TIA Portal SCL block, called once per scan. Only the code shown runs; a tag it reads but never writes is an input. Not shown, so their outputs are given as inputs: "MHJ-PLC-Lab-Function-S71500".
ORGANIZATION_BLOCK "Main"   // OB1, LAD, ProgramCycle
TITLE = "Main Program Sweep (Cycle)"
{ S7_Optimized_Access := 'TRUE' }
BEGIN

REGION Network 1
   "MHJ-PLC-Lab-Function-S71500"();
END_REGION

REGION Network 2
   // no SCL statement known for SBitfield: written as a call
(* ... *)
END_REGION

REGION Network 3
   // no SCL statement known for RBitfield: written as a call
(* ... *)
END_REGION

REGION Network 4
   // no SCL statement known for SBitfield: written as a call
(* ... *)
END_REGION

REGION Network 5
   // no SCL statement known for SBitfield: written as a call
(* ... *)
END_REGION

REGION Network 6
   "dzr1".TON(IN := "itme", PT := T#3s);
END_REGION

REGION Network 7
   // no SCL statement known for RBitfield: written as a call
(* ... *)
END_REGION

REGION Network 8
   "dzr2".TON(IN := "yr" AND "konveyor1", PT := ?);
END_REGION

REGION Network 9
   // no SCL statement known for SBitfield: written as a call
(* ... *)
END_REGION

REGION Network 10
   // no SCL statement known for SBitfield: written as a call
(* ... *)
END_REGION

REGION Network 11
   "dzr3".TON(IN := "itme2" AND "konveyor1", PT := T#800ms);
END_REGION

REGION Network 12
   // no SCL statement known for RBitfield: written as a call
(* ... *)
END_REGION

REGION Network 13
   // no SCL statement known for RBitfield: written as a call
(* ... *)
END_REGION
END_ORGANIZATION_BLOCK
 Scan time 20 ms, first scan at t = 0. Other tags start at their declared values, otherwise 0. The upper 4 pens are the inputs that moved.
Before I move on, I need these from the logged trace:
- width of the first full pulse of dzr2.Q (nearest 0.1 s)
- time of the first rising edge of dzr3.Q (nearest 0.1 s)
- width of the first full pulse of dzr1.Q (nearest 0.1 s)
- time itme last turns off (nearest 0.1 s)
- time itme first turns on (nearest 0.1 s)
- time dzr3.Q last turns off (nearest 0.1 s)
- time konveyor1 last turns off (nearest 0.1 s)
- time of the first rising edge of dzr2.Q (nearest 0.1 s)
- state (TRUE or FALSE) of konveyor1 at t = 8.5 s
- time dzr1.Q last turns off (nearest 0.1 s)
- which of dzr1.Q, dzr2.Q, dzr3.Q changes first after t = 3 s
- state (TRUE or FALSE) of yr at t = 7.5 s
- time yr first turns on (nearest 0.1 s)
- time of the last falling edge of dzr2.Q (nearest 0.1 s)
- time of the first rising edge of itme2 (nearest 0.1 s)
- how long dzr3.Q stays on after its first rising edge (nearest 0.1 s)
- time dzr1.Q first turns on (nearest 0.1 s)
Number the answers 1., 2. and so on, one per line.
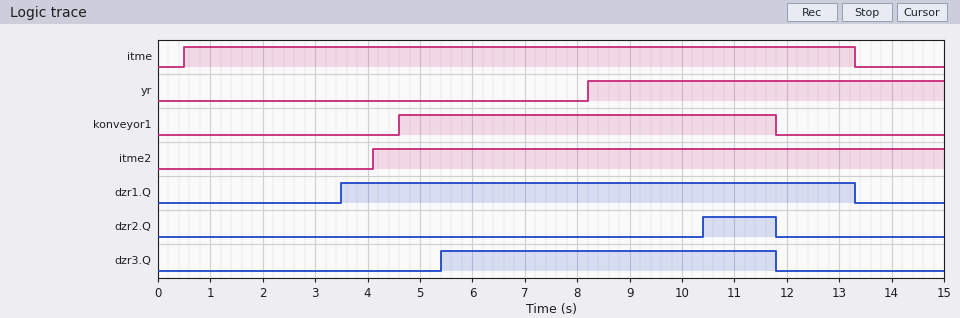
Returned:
1. 1.4 s
2. 5.4 s
3. 9.8 s
4. 13.3 s
5. 0.5 s
6. 11.8 s
7. 11.8 s
8. 10.4 s
9. TRUE
10. 13.3 s
11. dzr1.Q
12. FALSE
13. 8.2 s
14. 11.8 s
15. 4.1 s
16. 6.4 s
17. 3.5 s
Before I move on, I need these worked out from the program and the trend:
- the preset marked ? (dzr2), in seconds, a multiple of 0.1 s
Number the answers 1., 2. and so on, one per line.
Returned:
1. 2.2 s
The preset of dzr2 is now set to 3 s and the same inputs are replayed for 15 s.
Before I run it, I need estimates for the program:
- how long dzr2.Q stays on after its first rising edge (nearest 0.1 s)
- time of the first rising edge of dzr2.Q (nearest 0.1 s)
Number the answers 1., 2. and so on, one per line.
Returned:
1. 0.6 s
2. 11.2 s
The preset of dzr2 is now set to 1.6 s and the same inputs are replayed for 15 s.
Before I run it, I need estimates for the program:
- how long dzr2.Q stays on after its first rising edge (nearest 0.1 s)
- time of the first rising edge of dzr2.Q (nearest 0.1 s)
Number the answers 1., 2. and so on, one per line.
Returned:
1. 2.0 s
2. 9.8 s
